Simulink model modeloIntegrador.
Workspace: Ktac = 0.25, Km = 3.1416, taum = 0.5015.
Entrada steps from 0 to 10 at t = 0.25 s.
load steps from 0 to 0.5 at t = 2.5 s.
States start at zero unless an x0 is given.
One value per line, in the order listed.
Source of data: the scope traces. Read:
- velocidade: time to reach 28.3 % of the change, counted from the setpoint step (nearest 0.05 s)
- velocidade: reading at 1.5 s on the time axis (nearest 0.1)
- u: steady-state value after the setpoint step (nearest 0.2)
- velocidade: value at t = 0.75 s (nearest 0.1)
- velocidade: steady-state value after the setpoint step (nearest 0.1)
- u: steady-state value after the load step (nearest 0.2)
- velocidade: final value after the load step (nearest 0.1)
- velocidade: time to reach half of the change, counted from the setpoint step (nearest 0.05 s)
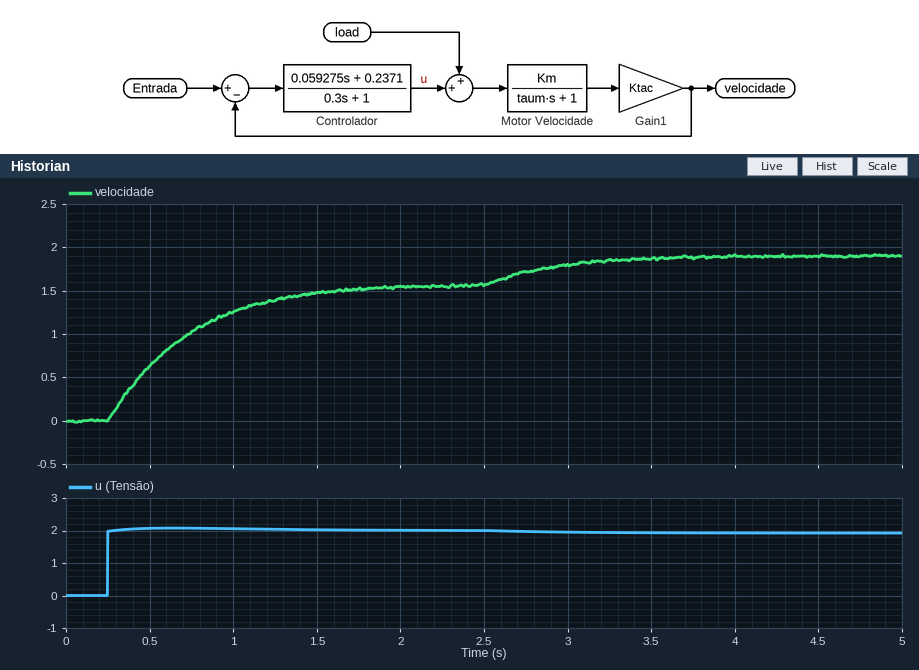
0.15 s
1.5
2.0
1.0
1.6
2.0
1.9
0.35 s
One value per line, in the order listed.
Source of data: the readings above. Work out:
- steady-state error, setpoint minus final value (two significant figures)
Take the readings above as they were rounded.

8.4
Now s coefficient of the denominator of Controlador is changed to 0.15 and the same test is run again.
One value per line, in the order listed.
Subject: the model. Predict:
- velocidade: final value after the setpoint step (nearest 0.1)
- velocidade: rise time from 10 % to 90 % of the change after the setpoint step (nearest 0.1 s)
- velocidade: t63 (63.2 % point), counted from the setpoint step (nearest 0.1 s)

1.6
0.8 s
0.3 s
